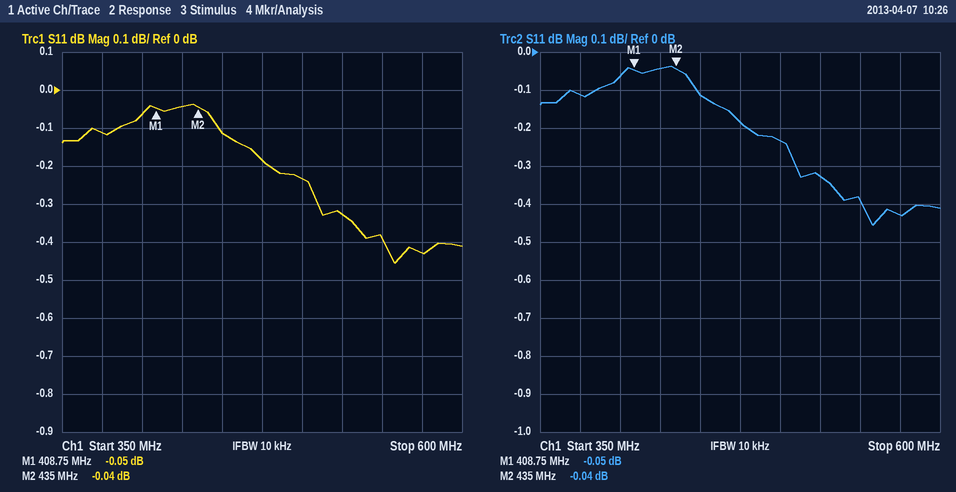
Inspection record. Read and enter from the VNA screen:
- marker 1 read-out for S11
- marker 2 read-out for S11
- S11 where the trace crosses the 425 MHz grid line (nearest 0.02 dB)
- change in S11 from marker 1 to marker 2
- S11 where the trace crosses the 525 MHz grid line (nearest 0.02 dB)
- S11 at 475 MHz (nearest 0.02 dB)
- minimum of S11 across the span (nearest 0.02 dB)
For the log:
-0.05 dB
-0.04 dB
-0.04 dB
0.01 dB
-0.32 dB
-0.18 dB
-0.46 dB
